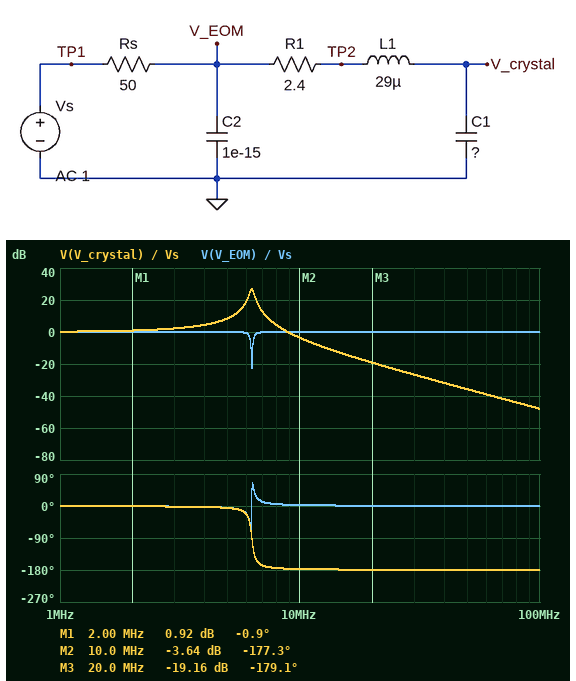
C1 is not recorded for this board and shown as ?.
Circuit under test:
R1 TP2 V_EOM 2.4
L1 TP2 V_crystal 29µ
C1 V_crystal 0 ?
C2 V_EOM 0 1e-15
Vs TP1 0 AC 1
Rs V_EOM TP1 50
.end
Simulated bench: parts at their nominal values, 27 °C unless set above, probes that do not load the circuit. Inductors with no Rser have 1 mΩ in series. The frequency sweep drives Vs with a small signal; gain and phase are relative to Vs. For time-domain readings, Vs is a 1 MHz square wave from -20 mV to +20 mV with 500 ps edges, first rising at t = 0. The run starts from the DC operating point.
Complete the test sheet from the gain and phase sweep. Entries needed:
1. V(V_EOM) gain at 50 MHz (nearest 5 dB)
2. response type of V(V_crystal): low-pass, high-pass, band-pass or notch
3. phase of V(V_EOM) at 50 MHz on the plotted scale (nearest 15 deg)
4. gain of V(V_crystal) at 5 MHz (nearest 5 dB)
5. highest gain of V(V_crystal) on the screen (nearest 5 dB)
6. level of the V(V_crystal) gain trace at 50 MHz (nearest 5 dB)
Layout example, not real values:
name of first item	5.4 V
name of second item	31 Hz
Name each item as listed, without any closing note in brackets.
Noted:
V(V_EOM) gain at 50 MHz	0 dB
response type of V(V_crystal): low-pass, high-pass, band-pass or notch	low-pass
phase of V(V_EOM) at 50 MHz on the plotted scale	0 deg
gain of V(V_crystal) at 5 MHz	10 dB
highest gain of V(V_crystal) on the screen	25 dB
level of the V(V_crystal) gain trace at 50 MHz	-35 dB
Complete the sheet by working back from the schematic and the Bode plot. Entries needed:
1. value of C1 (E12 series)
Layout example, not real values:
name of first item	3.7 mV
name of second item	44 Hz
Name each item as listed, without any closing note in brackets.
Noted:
value of C1	22 pF
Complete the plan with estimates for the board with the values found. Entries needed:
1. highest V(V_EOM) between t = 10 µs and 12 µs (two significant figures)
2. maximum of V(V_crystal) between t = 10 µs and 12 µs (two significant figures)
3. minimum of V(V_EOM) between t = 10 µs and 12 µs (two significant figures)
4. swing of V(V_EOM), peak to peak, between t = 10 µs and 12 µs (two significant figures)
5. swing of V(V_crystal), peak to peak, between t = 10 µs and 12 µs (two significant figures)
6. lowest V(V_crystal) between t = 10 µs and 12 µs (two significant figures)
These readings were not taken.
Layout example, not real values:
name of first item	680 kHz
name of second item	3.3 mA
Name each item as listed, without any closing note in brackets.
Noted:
highest V(V_EOM) between t = 10 µs and 12 µs	21 mV
maximum of V(V_crystal) between t = 10 µs and 12 µs	45 mV
minimum of V(V_EOM) between t = 10 µs and 12 µs	-21 mV
swing of V(V_EOM), peak to peak, between t = 10 µs and 12 µs	42 mV
swing of V(V_crystal), peak to peak, between t = 10 µs and 12 µs	90 mV
lowest V(V_crystal) between t = 10 µs and 12 µs	-45 mV
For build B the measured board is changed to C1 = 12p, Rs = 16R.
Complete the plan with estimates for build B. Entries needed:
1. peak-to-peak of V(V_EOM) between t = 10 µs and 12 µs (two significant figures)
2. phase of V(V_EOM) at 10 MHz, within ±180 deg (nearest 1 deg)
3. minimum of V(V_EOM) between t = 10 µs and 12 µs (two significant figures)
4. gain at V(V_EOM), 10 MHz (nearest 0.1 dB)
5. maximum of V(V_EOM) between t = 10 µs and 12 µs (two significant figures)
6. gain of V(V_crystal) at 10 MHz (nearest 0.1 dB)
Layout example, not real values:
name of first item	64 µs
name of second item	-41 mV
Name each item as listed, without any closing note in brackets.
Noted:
peak-to-peak of V(V_EOM) between t = 10 µs and 12 µs	41 mV
phase of V(V_EOM) at 10 MHz, within ±180 deg	2 deg
minimum of V(V_EOM) between t = 10 µs and 12 µs	-20 mV
gain at V(V_EOM), 10 MHz	0 dB
maximum of V(V_EOM) between t = 10 µs and 12 µs	20 mV
gain of V(V_crystal) at 10 MHz	8.5 dB
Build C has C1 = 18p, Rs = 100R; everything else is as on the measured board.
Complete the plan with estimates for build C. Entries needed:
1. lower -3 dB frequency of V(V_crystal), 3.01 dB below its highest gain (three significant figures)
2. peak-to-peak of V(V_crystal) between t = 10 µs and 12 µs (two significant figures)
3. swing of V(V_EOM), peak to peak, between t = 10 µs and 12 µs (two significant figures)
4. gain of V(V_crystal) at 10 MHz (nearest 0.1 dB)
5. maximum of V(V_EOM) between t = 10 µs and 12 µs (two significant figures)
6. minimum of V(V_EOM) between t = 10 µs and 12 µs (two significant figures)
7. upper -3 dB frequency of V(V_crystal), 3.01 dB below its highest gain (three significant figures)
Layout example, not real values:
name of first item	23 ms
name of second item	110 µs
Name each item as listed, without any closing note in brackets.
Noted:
lower -3 dB frequency of V(V_crystal), 3.01 dB below its highest gain	6.67 MHz
peak-to-peak of V(V_crystal) between t = 10 µs and 12 µs	160 mV
swing of V(V_EOM), peak to peak, between t = 10 µs and 12 µs	49 mV
gain of V(V_crystal) at 10 MHz	-0.6 dB
maximum of V(V_EOM) between t = 10 µs and 12 µs	24 mV
minimum of V(V_EOM) between t = 10 µs and 12 µs	-24 mV
upper -3 dB frequency of V(V_crystal), 3.01 dB below its highest gain	7.23 MHz
